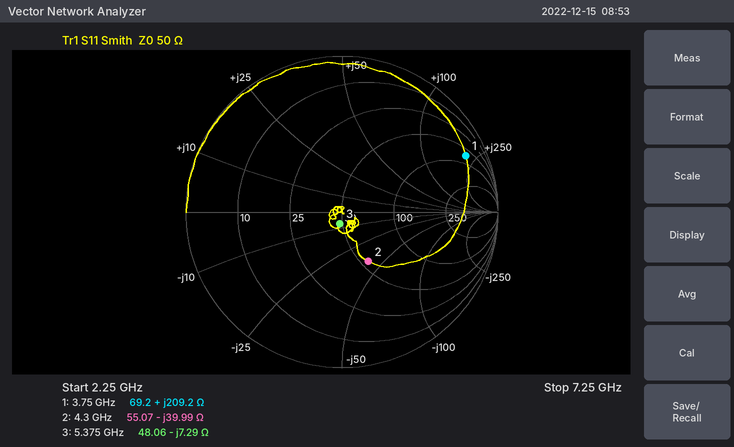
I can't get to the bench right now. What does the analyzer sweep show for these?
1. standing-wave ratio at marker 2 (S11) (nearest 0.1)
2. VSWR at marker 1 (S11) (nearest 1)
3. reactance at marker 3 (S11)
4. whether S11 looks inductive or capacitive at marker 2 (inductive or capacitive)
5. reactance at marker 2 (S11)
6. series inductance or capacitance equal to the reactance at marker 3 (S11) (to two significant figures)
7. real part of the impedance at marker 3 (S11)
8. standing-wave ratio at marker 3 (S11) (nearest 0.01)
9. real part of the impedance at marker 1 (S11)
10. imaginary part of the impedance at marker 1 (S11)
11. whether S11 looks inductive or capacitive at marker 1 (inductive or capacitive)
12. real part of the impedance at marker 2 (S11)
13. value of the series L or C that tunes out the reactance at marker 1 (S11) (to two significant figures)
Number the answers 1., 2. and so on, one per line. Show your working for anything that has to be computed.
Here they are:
1. 2.1
2. 15
3. -7.29 Ω
4. capacitive
5. -39.99 Ω
6. C = 1/(2π × 5.375 GHz × 7.29 Ω) ≈ 4.1 pF
7. 48.06 Ω
8. 1.17
9. 69.2 Ω
10. +209.2 Ω
11. inductive
12. 55.07 Ω
13. C = 1/(2π × 3.75 GHz × 209.2 Ω) ≈ 203 fF, so 200 fF to two significant figures
